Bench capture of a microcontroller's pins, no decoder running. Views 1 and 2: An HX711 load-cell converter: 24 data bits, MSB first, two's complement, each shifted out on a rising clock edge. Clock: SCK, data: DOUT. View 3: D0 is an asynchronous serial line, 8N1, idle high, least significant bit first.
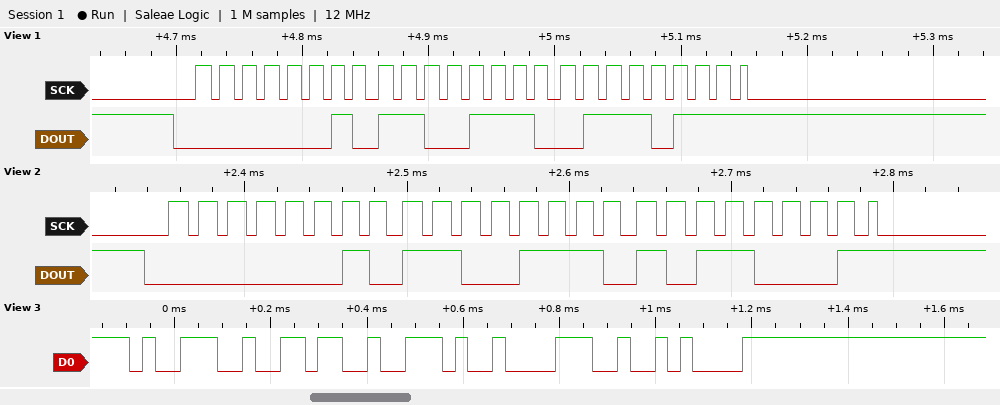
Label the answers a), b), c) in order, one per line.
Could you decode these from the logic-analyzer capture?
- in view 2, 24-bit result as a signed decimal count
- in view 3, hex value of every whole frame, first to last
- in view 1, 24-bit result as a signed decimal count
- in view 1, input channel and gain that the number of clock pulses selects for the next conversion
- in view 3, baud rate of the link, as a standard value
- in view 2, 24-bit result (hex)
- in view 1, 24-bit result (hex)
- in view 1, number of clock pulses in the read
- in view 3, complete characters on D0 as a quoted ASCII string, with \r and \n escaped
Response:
a) 183985
b) 0x39 0x36 0x2E 0x38 0x0A
c) 183927
d) channel A, gain 128
e) 38400 baud
f) 0x02CEB1
g) 0x02CE77
h) 25
i) "96.8\n"
